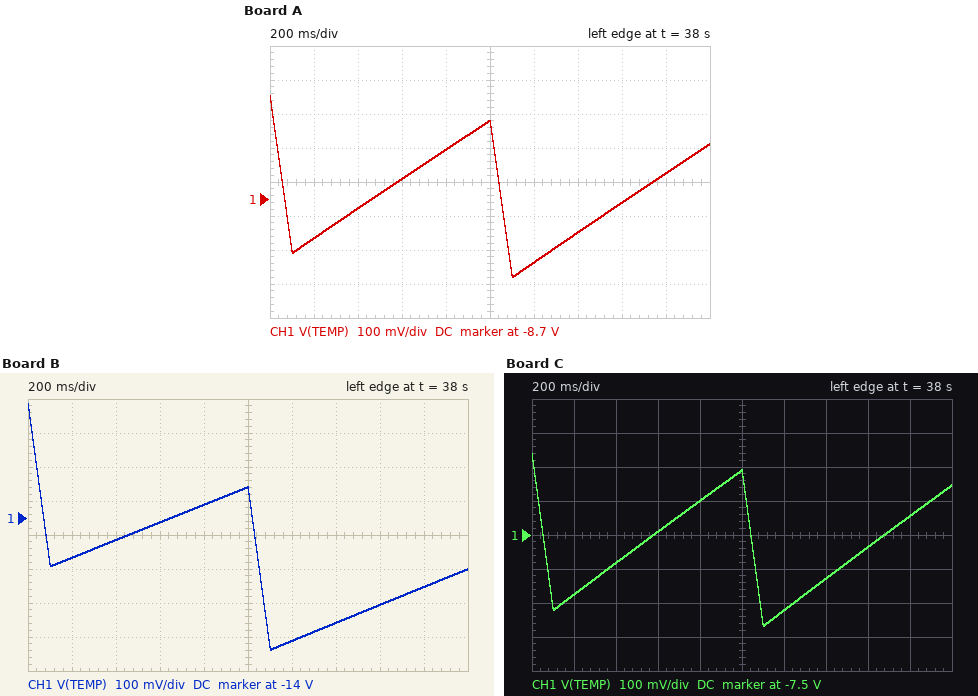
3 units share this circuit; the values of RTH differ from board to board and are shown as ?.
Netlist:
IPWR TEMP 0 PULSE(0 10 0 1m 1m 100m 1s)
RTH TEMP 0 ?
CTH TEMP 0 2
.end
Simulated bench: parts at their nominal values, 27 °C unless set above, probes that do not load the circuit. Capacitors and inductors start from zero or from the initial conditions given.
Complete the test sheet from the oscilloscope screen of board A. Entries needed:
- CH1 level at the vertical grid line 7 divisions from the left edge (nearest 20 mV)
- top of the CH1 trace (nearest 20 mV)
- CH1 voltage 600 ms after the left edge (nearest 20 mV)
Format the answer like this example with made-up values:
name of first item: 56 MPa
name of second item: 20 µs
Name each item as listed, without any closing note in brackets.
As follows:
CH1 level at the vertical grid line 7 divisions from the left edge: -8.80 V
top of the CH1 trace: -8.40 V
CH1 voltage 600 ms after the left edge: -8.64 V
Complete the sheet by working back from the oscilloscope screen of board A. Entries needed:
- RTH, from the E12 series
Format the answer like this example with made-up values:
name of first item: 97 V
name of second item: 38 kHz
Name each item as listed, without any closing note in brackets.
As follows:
RTH, from the E12 series: 10 Ω
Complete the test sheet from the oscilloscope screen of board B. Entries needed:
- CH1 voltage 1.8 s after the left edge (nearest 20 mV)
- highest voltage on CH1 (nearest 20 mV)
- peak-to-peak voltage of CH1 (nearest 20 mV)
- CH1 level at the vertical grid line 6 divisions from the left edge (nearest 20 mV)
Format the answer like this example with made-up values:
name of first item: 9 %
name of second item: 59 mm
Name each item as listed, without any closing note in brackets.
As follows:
CH1 voltage 1.8 s after the left edge: -14.20 V
highest voltage on CH1: -13.66 V
peak-to-peak voltage of CH1: 720 mV
CH1 level at the vertical grid line 6 divisions from the left edge: -14.36 V
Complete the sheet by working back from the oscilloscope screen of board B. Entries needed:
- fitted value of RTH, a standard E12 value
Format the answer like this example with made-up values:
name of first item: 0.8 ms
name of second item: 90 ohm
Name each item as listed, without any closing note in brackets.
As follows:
fitted value of RTH, a standard E12 value: 27 Ω
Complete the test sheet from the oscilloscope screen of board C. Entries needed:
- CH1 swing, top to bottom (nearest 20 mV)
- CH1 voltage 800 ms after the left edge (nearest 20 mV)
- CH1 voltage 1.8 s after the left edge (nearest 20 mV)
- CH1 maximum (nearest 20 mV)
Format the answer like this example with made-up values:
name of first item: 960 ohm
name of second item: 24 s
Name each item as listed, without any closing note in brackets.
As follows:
CH1 swing, top to bottom: 500 mV
CH1 voltage 800 ms after the left edge: -7.40 V
CH1 voltage 1.8 s after the left edge: -7.44 V
CH1 maximum: -7.26 V
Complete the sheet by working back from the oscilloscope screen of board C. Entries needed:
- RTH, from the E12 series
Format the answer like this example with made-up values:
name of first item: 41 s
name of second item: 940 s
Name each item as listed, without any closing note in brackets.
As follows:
RTH, from the E12 series: 8.2 Ω
